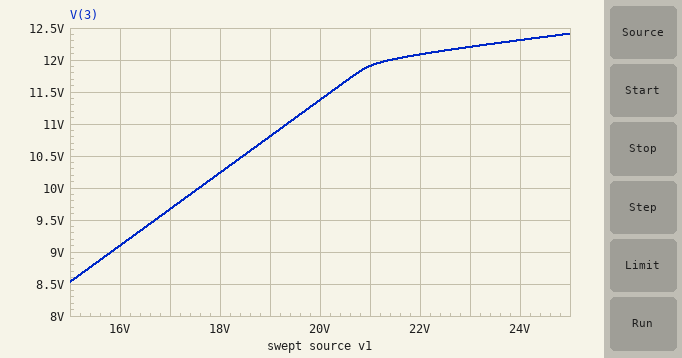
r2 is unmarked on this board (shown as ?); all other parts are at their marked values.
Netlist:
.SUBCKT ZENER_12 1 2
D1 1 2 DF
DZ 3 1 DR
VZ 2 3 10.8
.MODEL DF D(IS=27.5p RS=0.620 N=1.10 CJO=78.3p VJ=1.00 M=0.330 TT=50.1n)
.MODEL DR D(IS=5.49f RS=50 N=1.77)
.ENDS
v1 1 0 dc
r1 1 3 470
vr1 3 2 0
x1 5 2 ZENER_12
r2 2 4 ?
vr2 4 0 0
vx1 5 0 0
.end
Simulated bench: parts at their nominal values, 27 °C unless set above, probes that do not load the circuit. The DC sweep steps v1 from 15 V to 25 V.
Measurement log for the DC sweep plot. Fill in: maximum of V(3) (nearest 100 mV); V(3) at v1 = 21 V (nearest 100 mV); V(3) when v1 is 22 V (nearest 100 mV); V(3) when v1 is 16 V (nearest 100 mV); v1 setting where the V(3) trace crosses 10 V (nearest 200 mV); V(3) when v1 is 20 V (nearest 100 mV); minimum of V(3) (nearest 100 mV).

12.4 V
11.9 V
12.1 V
9.1 V
17.6 V
11.4 V
8.5 V
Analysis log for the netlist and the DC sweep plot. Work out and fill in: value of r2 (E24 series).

620 Ω
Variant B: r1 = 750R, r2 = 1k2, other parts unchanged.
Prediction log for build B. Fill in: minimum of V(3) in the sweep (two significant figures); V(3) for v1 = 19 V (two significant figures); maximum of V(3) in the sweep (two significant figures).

9.2 V
12 V
12 V
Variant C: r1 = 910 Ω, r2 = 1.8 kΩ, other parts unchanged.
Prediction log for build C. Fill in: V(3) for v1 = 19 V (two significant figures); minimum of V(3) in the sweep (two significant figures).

12 V
10 V
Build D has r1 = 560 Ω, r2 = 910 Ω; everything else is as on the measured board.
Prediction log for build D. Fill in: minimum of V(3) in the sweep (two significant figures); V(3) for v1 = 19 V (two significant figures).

9.3 V
12 V
